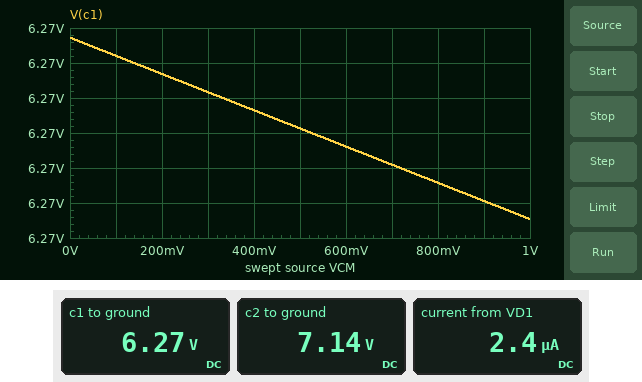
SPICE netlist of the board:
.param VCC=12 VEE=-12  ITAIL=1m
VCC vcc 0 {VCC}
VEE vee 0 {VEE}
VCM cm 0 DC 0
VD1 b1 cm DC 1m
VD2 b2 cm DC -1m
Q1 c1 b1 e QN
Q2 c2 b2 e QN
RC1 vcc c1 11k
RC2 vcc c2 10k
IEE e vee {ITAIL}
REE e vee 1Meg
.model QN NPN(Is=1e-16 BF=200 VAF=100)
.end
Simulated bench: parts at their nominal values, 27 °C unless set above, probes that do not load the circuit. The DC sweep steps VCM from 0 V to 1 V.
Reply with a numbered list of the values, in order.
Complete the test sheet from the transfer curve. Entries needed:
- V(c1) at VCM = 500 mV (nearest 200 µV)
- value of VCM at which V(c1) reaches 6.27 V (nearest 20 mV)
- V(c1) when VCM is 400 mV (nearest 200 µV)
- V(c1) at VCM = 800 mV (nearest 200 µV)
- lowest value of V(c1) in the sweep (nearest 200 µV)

1. 6.2702 V
2. 720 mV
3. 6.2706 V
4. 6.2686 V
5. 6.2676 V
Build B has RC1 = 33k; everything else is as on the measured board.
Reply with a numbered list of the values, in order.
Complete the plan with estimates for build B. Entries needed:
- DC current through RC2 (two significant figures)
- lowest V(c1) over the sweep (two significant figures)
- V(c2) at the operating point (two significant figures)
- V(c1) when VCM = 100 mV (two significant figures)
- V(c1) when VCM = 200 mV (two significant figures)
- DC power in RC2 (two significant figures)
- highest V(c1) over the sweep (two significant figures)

1. 540 µA
2. -710 mV
3. 6.6 V
4. -610 mV
5. -510 mV
6. 2.9 mW
7. 290 mV
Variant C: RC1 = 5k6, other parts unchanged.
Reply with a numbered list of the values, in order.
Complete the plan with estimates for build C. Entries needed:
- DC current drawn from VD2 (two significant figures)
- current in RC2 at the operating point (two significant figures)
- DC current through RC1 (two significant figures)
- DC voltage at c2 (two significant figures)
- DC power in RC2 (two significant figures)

1. 2.2 µA
2. 480 µA
3. 530 µA
4. 7.2 V
5. 2.3 mW
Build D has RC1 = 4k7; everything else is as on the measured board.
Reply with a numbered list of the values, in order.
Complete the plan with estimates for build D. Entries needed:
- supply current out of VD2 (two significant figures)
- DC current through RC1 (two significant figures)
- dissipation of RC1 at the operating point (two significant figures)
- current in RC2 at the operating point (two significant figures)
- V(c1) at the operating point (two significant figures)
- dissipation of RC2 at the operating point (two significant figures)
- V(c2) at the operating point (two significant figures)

1. 2.2 µA
2. 530 µA
3. 1.3 mW
4. 480 µA
5. 9.5 V
6. 2.3 mW
7. 7.2 V
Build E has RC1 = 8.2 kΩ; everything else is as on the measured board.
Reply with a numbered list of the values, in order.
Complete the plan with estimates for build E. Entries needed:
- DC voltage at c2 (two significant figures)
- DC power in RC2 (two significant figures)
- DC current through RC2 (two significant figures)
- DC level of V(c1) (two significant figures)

1. 7.2 V
2. 2.3 mW
3. 480 µA
4. 7.7 V
